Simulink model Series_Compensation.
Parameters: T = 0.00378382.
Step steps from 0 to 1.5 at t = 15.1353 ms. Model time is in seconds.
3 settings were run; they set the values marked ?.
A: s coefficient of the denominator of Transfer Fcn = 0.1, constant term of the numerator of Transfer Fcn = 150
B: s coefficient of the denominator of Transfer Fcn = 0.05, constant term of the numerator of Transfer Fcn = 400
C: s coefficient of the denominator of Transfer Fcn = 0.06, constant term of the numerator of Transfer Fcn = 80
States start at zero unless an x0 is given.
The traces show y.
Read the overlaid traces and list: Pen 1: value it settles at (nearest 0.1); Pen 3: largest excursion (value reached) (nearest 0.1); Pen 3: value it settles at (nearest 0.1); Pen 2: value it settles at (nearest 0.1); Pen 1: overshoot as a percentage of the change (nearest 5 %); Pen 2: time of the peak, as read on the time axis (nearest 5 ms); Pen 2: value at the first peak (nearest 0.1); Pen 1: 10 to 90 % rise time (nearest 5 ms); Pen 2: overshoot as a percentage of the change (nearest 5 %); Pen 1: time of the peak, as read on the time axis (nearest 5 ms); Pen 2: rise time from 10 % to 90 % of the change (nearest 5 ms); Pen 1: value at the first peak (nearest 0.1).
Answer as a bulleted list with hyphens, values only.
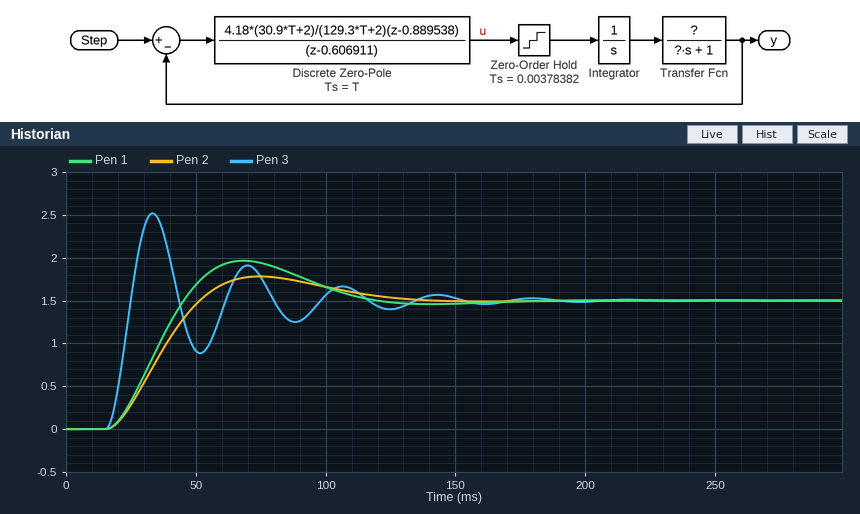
- 1.5
- 2.5
- 1.5
- 1.5
- 30 %
- 75 ms
- 1.8
- 20 ms
- 20 %
- 70 ms
- 25 ms
- 2.0
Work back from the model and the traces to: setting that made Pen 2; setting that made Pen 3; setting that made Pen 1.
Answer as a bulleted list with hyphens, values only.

- C
- B
- A
